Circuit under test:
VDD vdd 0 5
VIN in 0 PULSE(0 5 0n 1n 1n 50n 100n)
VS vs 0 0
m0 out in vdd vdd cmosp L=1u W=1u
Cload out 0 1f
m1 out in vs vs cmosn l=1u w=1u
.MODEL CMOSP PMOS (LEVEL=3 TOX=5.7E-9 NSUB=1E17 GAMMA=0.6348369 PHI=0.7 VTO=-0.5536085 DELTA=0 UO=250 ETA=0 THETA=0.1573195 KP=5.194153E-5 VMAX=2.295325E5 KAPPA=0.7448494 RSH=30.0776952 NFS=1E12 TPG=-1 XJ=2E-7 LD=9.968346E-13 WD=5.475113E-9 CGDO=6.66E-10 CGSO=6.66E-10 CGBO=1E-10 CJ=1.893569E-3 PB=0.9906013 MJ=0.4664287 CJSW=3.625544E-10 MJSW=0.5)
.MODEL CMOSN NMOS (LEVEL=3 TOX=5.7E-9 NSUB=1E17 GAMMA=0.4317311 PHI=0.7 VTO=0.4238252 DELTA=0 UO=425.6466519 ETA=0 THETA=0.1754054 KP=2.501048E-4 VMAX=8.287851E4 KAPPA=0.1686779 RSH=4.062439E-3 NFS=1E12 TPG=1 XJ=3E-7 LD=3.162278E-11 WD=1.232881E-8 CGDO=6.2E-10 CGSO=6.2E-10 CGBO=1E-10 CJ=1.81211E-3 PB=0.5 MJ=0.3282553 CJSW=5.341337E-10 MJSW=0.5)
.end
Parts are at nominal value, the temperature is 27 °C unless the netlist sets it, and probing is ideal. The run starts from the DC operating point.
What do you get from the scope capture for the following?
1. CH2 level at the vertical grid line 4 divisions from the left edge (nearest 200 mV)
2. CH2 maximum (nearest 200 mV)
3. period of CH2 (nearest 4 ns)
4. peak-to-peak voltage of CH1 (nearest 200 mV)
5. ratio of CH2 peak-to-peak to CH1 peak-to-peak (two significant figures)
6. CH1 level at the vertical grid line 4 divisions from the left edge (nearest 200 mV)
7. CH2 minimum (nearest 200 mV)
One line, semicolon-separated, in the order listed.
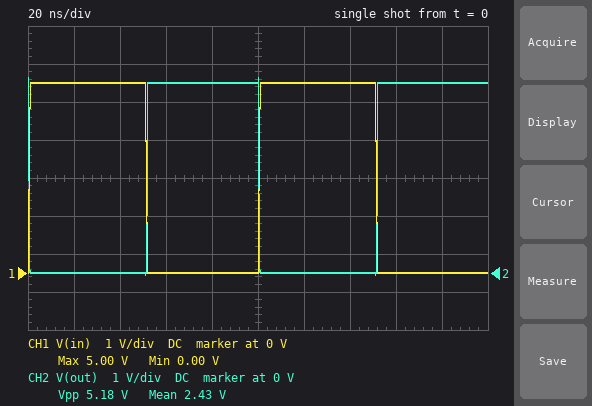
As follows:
5.0 V; 5.2 V; 100 ns; 5.0 V; 1.0; 0 V; 0 V
